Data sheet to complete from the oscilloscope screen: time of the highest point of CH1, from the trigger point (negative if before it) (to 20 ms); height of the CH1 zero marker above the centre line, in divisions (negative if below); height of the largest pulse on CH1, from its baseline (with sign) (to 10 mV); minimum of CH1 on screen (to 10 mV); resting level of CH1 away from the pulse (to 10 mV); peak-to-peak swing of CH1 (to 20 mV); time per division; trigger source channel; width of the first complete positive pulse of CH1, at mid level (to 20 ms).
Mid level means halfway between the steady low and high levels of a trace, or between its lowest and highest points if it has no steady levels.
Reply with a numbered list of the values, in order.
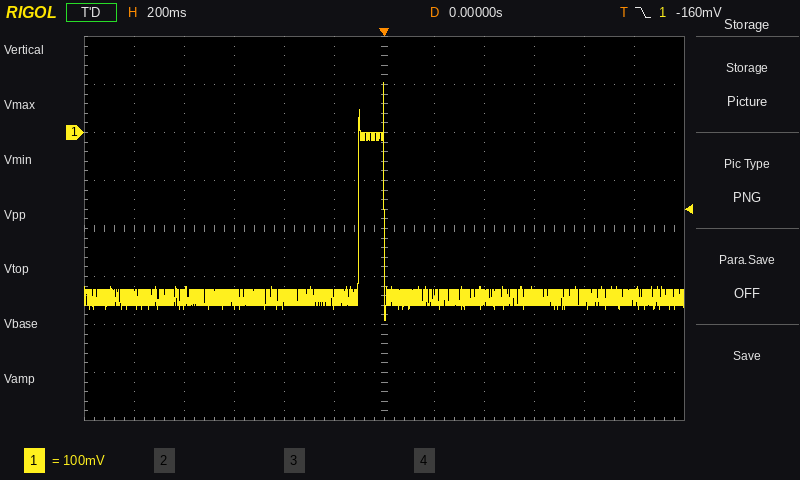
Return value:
1. 0 ms
2. +2.0 div
3. +450 mV
4. -390 mV
5. -340 mV
6. 500 mV
7. 200 ms
8. CH1
9. 100 ms
